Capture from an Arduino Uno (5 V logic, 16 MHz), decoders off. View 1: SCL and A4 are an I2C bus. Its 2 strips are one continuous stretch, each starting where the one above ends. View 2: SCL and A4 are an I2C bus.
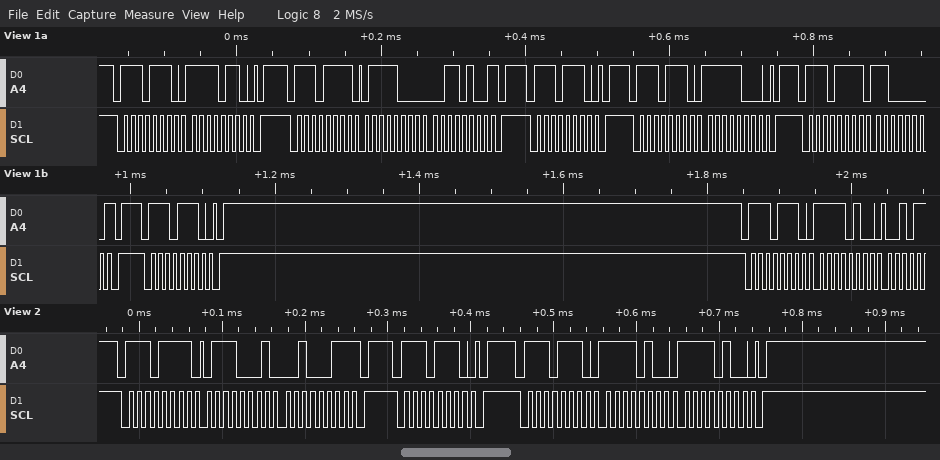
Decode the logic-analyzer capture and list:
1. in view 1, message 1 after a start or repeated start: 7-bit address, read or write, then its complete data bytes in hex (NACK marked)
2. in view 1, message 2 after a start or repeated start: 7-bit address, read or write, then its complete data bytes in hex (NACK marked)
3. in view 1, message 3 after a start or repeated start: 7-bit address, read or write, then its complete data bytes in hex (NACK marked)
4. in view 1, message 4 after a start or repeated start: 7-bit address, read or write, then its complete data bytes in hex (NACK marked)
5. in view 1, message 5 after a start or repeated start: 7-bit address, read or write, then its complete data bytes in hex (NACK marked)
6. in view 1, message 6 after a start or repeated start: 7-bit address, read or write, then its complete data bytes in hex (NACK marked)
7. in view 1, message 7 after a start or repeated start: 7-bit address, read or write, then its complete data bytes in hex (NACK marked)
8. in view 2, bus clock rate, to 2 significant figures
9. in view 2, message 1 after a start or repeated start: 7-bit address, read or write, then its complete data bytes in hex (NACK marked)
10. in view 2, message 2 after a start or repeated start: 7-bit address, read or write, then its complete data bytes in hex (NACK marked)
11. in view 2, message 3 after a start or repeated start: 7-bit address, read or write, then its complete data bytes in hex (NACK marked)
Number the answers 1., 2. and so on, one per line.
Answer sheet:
1. 0x77 write: F6
2. 0x77 read: 78 34 NACK
3. 0x77 write
4. 0x77 write: F8
5. 0x77 read: C0 NACK
6. 0x77 write
7. 0x77 write: F4
8. 100 kHz
9. 0x77 read: 71 23 NACK
10. 0x77 write
11. 0x77 write: F4 F4
